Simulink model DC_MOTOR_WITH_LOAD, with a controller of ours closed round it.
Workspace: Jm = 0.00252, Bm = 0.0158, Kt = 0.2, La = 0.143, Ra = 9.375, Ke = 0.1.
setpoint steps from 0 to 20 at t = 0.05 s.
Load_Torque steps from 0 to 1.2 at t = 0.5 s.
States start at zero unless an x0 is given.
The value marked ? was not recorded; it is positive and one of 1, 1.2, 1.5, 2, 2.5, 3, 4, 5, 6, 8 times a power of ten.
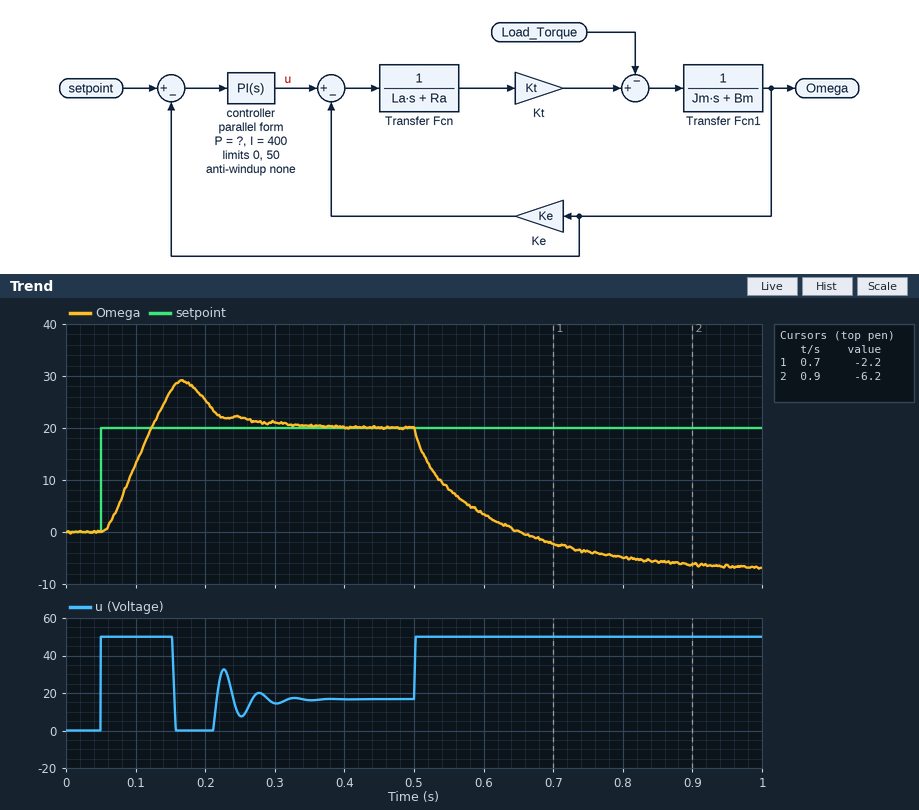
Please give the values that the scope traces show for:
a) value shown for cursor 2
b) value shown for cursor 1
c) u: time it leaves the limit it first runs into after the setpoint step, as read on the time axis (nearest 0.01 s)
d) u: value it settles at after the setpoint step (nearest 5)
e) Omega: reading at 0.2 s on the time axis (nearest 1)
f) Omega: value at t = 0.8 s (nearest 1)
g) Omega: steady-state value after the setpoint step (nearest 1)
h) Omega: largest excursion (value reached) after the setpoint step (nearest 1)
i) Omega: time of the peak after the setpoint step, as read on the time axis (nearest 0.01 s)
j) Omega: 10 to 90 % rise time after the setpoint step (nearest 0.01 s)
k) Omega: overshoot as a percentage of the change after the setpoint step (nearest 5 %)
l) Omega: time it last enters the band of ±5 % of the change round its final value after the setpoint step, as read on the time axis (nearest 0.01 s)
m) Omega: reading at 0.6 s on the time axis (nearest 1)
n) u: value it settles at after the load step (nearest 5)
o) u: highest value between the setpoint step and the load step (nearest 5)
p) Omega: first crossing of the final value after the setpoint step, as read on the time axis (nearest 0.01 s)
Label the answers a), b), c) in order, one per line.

a) -6.2
b) -2.2
c) 0.15 s
d) 15
e) 25
f) -5
g) 20
h) 29
i) 0.17 s
j) 0.05 s
k) 45 %
l) 0.30 s
m) 3
n) 50
o) 50
p) 0.12 s
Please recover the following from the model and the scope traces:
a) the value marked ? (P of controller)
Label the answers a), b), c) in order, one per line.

a) 30
